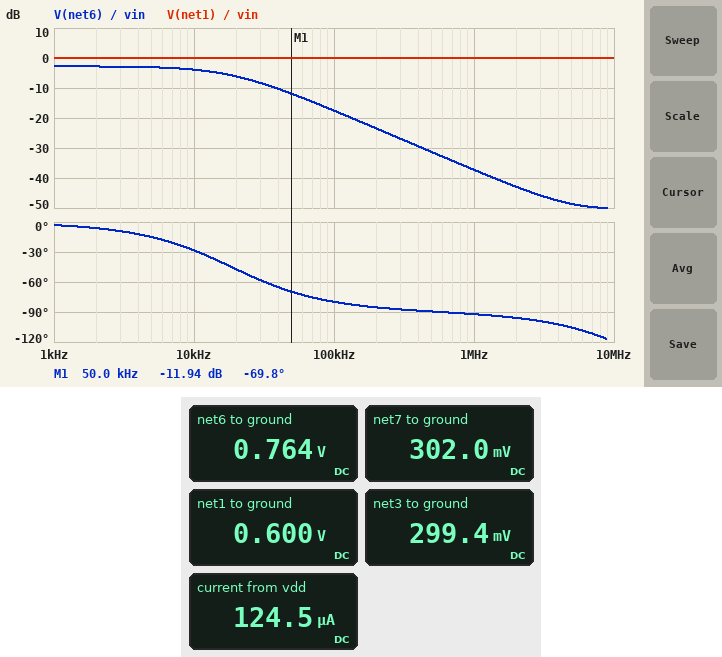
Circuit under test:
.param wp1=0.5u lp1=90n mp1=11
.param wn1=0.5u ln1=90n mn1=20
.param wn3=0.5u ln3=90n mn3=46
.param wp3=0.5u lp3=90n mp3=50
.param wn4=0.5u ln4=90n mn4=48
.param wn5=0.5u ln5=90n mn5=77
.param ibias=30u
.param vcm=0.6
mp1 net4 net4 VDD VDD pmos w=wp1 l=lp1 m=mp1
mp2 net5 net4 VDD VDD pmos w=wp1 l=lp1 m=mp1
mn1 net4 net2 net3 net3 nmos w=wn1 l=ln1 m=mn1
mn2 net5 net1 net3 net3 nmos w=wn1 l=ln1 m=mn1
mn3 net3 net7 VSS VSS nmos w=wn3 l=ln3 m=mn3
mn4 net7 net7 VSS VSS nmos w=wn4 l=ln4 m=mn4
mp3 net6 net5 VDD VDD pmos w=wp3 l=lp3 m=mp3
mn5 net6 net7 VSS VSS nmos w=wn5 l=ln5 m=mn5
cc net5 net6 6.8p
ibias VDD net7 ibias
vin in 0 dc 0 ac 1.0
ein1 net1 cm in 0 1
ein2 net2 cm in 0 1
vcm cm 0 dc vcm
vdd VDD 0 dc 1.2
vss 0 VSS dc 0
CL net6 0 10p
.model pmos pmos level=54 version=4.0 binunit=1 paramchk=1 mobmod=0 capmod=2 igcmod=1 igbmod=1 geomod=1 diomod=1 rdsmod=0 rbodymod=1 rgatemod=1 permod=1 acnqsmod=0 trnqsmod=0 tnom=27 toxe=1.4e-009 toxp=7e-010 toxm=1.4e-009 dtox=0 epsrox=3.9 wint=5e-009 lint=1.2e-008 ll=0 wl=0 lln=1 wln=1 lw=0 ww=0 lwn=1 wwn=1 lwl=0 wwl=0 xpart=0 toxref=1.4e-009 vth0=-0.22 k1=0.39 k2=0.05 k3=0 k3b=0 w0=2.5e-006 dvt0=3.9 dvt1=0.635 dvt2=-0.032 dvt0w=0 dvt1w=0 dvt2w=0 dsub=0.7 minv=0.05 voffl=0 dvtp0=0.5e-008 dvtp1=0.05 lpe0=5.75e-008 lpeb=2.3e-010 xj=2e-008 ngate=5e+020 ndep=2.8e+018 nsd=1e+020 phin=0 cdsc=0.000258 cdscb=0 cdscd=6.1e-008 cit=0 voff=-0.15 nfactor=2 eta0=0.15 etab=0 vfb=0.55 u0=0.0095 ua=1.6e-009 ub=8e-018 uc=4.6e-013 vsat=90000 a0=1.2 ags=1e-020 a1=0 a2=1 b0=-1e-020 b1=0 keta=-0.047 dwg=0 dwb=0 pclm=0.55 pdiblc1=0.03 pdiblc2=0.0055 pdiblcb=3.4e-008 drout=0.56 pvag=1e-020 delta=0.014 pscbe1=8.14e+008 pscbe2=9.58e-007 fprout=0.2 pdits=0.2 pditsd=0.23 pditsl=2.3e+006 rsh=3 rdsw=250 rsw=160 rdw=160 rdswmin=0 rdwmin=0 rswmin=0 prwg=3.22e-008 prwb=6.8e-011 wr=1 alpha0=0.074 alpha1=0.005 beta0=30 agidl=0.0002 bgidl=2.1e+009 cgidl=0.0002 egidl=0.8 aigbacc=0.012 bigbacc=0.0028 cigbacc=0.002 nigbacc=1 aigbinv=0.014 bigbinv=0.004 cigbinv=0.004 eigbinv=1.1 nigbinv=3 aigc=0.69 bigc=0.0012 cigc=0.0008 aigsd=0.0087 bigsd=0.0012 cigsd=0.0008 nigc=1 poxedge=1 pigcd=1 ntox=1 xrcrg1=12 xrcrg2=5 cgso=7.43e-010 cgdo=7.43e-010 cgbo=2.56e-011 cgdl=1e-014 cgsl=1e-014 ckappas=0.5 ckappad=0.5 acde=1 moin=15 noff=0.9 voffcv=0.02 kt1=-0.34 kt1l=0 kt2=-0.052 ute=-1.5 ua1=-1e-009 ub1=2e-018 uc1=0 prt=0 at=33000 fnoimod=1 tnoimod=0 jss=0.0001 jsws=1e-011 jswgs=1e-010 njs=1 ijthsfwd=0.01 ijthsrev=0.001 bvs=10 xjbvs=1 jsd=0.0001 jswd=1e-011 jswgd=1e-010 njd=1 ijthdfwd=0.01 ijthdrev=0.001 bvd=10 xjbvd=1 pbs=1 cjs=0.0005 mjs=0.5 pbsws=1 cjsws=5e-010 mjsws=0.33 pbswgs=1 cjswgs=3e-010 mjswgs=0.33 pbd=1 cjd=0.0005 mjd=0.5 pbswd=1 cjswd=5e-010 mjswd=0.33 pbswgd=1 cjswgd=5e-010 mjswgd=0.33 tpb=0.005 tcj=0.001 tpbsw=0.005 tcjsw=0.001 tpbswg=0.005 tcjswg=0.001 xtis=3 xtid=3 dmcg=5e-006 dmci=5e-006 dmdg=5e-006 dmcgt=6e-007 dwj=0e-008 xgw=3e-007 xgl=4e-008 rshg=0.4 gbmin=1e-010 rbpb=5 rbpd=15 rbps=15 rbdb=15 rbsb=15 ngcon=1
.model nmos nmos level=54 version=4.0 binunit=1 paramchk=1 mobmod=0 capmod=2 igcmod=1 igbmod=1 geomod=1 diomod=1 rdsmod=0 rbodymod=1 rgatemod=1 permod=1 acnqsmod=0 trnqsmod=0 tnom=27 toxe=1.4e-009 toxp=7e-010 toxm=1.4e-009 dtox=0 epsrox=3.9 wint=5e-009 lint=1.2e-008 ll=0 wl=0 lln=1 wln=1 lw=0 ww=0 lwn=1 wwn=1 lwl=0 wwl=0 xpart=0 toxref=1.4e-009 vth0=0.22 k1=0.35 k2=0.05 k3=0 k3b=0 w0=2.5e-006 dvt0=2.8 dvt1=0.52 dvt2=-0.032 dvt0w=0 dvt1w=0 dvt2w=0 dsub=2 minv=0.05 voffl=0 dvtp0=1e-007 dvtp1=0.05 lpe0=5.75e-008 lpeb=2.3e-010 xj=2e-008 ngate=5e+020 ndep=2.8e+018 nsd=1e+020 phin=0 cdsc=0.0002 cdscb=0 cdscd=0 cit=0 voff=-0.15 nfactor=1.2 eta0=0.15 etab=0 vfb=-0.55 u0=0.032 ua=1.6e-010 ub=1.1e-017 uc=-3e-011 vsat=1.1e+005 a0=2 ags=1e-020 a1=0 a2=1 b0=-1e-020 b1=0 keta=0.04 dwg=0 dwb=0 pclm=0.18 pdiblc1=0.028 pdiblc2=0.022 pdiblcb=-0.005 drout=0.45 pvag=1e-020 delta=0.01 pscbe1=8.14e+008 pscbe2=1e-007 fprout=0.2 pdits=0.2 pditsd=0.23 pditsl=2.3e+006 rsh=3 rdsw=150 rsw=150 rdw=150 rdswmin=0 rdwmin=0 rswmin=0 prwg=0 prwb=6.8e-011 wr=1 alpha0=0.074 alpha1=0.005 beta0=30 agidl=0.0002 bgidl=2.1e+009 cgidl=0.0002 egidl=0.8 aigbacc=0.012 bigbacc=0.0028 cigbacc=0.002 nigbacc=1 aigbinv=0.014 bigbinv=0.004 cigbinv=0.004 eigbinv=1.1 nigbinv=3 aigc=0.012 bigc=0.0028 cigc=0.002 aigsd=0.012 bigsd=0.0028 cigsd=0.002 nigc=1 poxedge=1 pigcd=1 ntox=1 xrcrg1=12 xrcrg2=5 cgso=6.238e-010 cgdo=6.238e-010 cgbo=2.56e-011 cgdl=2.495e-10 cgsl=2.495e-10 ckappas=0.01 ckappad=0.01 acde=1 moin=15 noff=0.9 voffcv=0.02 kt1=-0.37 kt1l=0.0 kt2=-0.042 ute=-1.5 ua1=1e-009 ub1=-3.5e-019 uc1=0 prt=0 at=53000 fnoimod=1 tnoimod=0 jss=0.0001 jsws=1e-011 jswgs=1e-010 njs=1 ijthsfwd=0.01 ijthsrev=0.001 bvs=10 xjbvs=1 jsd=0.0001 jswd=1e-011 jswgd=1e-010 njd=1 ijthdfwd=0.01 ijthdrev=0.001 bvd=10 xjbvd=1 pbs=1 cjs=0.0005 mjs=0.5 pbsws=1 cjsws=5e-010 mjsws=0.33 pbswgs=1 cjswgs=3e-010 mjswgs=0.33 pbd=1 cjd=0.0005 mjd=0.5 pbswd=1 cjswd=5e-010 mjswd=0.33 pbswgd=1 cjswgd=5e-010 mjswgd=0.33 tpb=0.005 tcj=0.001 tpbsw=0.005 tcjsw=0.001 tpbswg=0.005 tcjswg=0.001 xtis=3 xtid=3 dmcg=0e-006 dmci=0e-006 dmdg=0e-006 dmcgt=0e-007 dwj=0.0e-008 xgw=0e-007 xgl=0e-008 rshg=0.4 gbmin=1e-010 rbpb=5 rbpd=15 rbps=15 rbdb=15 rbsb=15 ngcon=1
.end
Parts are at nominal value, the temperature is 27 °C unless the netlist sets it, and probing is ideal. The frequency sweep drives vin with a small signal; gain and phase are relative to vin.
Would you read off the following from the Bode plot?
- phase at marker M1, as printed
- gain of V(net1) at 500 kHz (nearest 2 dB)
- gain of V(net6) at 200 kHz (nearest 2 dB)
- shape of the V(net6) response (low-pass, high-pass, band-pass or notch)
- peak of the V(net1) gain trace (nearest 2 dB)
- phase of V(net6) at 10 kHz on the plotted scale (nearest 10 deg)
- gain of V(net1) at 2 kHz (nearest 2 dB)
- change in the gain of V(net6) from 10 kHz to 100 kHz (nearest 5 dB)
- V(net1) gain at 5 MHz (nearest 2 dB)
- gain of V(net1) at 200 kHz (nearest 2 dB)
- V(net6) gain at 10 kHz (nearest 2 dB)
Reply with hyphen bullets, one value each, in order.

- -69.8 deg
- 0 dB
- -24 dB
- low-pass
- 0 dB
- -30 deg
- 0 dB
- -15 dB
- 0 dB
- 0 dB
- -4 dB
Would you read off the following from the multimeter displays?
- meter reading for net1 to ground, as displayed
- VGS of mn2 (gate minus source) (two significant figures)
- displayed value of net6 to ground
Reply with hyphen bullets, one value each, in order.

- 0.600 V
- 300 mV
- 0.764 V
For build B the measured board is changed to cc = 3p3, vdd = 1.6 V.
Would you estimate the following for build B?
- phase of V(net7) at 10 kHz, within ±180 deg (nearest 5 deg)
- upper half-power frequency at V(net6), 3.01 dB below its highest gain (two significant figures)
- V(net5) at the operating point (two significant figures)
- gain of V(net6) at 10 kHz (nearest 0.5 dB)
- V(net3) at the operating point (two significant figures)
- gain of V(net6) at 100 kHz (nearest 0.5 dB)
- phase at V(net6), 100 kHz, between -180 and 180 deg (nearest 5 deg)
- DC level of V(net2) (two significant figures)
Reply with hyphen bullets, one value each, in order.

- -15 deg
- 40 kHz
- 1.2 V
- -5.0 dB
- 310 mV
- -13.5 dB
- -70 deg
- 600 mV
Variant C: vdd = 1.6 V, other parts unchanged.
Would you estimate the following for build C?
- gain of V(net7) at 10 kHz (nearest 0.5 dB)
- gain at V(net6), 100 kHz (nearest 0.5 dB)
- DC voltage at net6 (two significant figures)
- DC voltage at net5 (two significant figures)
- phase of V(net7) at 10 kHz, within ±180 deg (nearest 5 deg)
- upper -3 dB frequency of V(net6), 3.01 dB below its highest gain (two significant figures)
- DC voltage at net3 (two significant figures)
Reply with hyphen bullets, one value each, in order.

- -45.0 dB
- -19.0 dB
- 930 mV
- 1.2 V
- -25 deg
- 20 kHz
- 310 mV
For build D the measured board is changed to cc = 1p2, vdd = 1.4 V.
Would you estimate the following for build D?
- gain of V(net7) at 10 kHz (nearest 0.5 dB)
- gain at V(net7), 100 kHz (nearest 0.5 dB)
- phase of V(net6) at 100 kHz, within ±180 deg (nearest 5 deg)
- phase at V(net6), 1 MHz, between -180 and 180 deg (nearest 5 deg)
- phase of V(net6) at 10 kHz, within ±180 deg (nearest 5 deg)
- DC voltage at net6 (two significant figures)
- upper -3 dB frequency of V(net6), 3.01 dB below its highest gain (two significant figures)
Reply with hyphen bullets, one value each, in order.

- -46.5 dB
- -49.5 dB
- -45 deg
- -85 deg
- -5 deg
- 840 mV
- 95 kHz
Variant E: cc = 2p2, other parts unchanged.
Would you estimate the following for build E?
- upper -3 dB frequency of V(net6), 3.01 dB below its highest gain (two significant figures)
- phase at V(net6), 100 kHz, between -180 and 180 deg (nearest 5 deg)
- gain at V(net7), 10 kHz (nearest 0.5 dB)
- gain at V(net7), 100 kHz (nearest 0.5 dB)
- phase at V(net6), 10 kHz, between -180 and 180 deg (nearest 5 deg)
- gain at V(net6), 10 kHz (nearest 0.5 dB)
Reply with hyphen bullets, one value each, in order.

- 55 kHz
- -60 deg
- -50.0 dB
- -56.0 dB
- -10 deg
- -3.0 dB
